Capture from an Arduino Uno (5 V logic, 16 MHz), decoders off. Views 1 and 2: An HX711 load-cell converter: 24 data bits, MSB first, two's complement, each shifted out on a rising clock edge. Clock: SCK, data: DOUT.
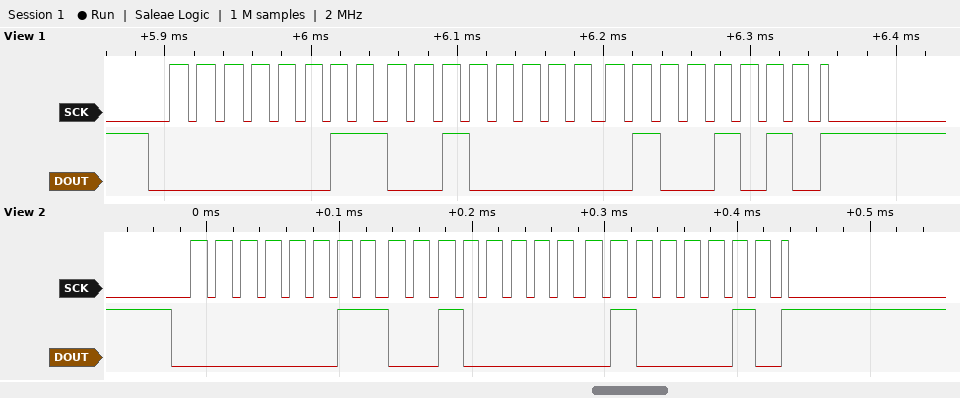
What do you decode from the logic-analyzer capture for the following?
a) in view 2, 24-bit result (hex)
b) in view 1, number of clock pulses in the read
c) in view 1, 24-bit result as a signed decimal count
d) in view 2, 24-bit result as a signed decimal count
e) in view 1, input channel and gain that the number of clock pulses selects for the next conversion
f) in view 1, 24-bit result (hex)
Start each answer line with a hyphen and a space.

- 0x032042
- 25
- 204874
- 204866
- channel A, gain 128
- 0x03204A
